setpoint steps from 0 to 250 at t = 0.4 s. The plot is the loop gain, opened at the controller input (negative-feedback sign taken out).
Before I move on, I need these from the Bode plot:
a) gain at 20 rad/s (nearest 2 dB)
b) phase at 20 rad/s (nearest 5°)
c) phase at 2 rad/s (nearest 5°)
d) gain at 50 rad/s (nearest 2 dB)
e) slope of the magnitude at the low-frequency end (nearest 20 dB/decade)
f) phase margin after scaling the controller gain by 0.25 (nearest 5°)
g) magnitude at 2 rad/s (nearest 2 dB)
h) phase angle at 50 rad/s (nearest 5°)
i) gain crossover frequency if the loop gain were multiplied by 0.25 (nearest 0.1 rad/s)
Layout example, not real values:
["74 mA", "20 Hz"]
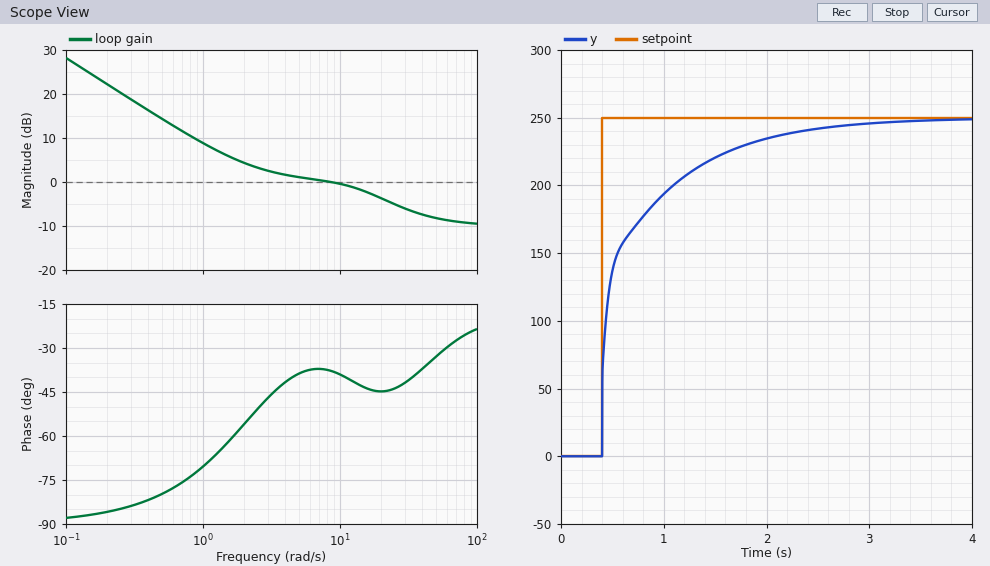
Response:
["-4 dB", "-45°", "-55°", "-8 dB", "-20 dB/decade", "105°", "4 dB", "-35°", "0.7 rad/s"]
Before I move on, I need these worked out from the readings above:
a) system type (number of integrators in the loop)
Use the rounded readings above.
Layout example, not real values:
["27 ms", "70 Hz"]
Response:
["1"]
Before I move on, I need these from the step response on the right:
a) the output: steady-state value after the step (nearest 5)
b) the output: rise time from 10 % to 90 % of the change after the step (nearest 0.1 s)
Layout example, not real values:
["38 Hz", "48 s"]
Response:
["250", "1.2 s"]
